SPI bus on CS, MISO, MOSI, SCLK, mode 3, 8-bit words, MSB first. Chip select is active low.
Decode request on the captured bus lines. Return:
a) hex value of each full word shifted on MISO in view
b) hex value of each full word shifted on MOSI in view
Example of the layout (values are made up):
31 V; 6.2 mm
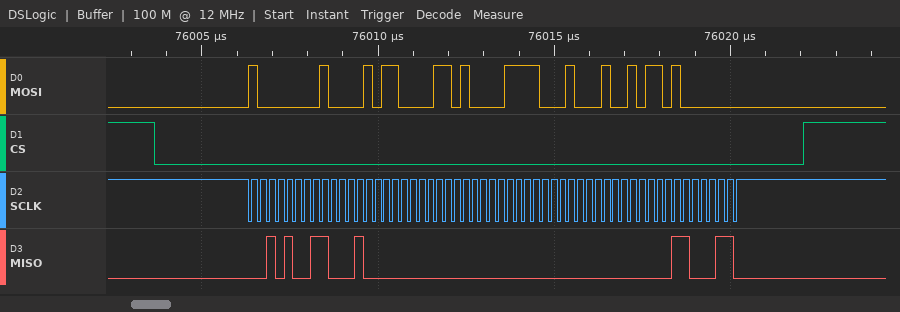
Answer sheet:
29, 88, 00, 00, 00, 00, C6; 80, 85, 86, 87, 88, 96, 80
